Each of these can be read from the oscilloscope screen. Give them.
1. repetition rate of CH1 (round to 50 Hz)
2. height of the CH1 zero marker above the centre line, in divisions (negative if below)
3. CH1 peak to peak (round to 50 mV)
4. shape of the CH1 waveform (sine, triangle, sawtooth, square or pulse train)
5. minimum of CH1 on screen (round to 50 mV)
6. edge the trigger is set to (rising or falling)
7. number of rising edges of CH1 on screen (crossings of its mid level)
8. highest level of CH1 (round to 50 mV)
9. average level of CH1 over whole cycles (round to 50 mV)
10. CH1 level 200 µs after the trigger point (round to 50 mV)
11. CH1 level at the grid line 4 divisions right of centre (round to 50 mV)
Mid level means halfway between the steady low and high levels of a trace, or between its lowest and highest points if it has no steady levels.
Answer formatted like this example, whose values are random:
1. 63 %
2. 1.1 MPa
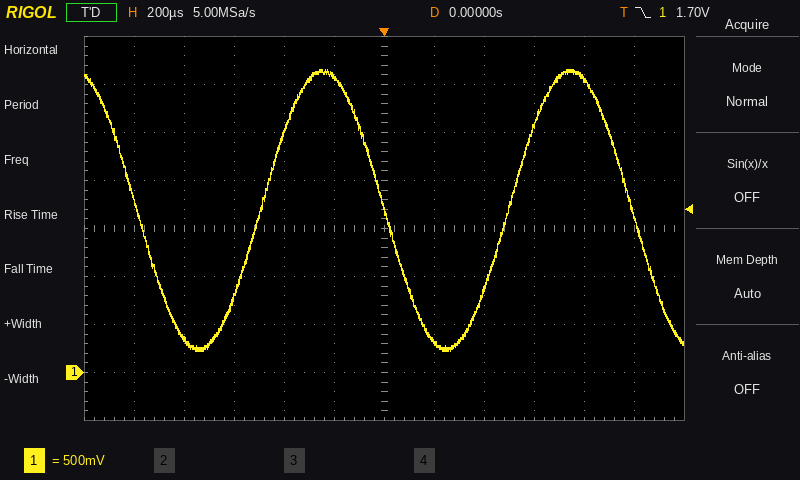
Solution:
1. 1.00 kHz
2. -3.0 div
3. 2.95 V
4. sine
5. 200 mV
6. falling
7. 2
8. 3.15 V
9. 1.70 V
10. 300 mV
11. 3.05 V
